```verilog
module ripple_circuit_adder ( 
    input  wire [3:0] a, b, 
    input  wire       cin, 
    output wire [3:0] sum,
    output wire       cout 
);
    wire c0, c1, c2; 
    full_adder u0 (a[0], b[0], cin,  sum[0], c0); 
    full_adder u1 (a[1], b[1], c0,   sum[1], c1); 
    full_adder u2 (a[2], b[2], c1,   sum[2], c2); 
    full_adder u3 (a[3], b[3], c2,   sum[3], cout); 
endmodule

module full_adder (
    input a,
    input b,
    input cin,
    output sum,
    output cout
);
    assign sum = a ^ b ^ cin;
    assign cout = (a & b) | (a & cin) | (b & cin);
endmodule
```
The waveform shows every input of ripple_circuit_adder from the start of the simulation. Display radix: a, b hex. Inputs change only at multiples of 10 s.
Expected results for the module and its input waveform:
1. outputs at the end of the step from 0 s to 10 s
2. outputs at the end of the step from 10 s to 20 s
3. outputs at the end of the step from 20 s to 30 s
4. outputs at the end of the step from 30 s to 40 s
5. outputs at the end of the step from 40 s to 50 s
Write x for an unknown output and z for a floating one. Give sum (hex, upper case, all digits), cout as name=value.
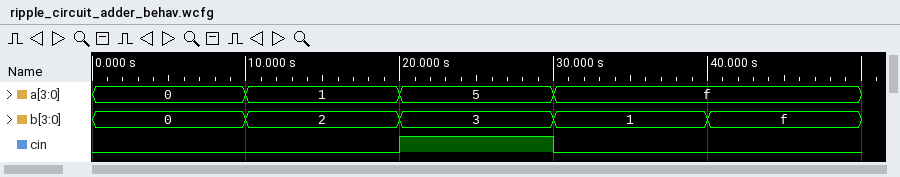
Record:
sum=0, cout=0
sum=3, cout=0
sum=9, cout=0
sum=0, cout=1
sum=E, cout=1
